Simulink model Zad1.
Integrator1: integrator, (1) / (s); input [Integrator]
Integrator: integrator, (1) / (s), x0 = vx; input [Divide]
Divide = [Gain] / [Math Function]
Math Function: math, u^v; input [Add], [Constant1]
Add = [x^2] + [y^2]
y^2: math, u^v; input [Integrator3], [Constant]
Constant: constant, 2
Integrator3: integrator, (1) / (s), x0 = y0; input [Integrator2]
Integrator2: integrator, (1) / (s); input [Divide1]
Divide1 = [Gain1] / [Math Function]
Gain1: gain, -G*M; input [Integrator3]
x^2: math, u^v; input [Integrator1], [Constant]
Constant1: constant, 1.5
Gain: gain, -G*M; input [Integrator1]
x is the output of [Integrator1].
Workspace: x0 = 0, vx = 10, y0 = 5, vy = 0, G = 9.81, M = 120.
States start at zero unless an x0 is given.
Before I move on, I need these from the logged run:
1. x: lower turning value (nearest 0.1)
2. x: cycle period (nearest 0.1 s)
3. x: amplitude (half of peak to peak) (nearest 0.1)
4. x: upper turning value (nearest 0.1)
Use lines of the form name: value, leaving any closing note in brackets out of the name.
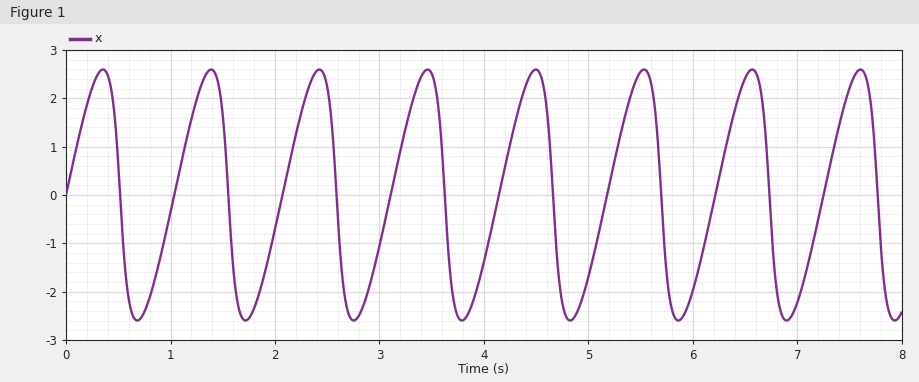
x: lower turning value: -2.6
x: cycle period: 1.0 s
x: amplitude (half of peak to peak): 2.6
x: upper turning value: 2.6
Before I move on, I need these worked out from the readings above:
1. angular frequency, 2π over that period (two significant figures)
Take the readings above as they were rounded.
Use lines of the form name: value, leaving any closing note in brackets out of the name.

angular frequency, 2π over that period: 6.3 rad/s
